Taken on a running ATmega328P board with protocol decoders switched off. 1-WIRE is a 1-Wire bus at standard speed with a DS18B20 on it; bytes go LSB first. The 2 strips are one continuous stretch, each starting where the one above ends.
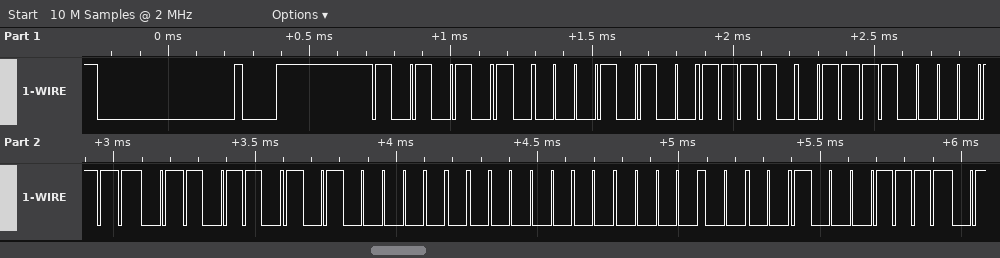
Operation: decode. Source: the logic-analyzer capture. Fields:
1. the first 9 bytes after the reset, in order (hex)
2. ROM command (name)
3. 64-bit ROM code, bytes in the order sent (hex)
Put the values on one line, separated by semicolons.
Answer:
55 28 CF C3 6D 05 00 00 F1; Match ROM; 28 CF C3 6D 05 00 00 F1
